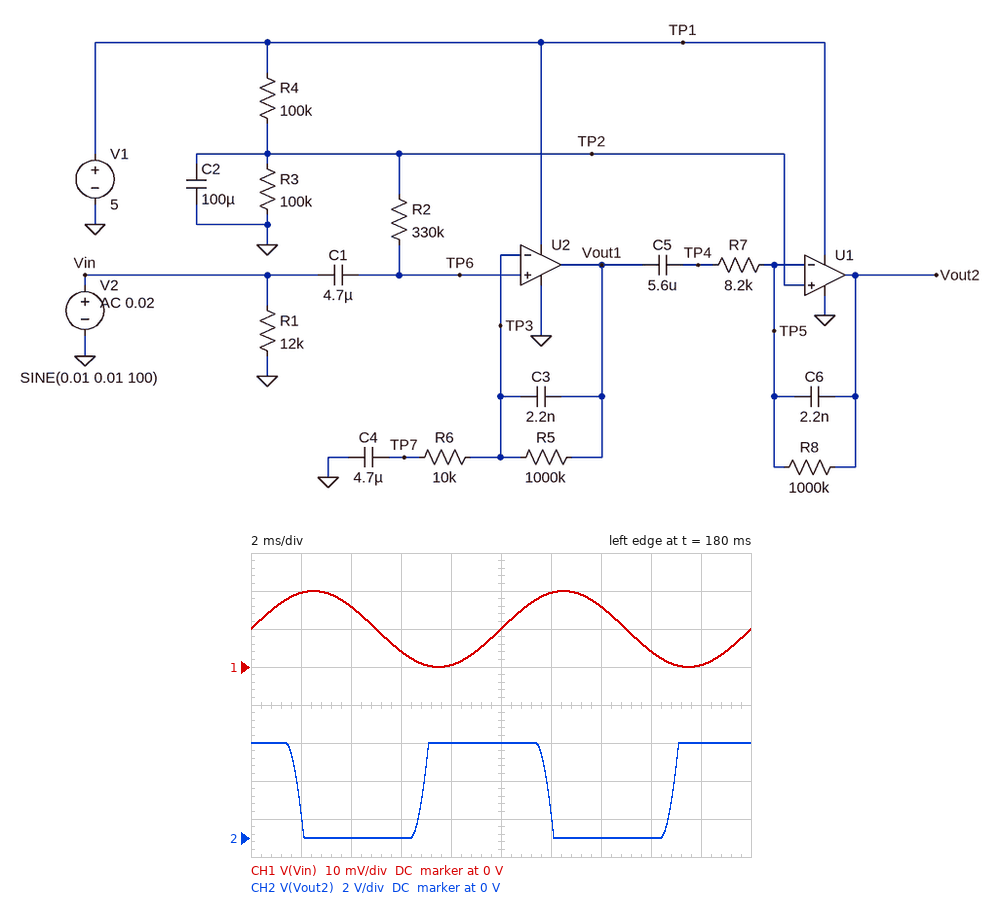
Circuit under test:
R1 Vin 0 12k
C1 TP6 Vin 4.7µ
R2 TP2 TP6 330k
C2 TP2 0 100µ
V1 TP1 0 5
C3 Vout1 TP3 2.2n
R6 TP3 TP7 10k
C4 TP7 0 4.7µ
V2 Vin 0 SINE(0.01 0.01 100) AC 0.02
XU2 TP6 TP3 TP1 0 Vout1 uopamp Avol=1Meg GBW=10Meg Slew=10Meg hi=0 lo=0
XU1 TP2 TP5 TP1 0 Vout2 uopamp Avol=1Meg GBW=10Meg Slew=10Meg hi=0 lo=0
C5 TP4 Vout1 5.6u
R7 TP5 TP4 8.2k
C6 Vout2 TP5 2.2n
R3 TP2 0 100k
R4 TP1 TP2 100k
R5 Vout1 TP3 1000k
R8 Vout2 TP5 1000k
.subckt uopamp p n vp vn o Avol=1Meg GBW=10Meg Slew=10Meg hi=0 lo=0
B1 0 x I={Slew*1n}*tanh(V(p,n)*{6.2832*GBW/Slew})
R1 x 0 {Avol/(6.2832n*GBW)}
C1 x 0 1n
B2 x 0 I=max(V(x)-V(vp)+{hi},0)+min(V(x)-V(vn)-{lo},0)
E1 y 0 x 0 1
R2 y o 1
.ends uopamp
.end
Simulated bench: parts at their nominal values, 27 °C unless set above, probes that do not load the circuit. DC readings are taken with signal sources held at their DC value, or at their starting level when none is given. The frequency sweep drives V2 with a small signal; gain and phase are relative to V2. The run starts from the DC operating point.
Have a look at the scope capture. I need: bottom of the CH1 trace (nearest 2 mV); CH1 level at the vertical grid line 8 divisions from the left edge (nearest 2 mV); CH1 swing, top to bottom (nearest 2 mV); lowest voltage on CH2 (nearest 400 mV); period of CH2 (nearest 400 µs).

0 V
4 mV
20 mV
0 V
10.0 ms
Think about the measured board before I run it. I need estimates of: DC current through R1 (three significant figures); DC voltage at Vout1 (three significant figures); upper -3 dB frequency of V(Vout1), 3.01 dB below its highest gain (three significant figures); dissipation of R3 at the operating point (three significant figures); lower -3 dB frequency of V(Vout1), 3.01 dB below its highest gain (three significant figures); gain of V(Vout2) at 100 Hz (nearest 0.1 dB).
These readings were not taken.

833 nA
2.50 V
78.8 Hz
62.5 µW
3.11 Hz
72.5 dB
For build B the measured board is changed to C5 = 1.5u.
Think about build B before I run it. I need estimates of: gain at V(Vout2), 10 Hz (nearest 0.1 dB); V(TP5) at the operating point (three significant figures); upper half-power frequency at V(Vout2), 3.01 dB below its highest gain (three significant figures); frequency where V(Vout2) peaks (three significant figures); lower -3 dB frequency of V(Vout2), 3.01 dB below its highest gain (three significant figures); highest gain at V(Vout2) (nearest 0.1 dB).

76.9 dB
2.50 V
63.0 Hz
25.5 Hz
9.69 Hz
79.7 dB
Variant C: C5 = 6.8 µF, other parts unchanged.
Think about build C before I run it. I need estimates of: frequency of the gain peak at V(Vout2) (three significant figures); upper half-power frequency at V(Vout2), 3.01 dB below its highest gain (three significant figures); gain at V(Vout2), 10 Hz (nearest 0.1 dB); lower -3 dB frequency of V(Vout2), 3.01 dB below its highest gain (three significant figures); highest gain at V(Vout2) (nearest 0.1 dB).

15.0 Hz
52.8 Hz
80.8 dB
4.28 Hz
81.1 dB
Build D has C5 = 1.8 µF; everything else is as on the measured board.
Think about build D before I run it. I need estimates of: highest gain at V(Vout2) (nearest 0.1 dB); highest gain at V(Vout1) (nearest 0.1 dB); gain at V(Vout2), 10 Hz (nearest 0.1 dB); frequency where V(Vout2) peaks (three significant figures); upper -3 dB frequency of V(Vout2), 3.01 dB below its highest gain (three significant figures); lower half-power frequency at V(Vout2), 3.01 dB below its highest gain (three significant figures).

80.0 dB
39.7 dB
77.8 dB
23.6 Hz
60.9 Hz
8.67 Hz
